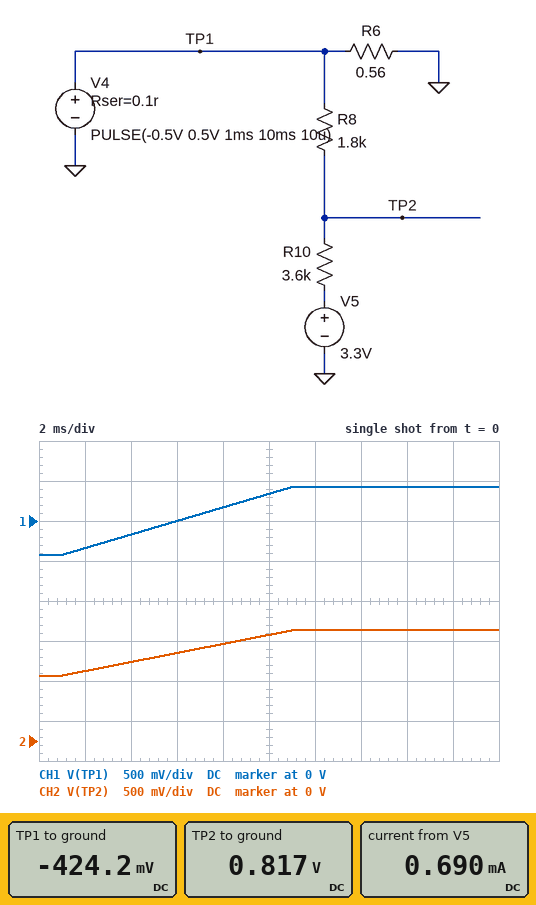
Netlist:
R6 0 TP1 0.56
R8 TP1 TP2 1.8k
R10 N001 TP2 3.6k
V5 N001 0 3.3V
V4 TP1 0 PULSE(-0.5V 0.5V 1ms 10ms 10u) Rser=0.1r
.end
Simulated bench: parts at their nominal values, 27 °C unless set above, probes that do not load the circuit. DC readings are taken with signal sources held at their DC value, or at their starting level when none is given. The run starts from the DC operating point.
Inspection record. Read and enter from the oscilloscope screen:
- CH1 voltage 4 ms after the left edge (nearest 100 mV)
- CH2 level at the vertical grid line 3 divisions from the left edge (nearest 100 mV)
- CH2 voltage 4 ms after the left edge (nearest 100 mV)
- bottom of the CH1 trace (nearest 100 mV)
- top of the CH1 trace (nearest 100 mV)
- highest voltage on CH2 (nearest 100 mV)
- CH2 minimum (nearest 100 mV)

-200 mV
1.1 V
1.0 V
-400 mV
400 mV
1.4 V
800 mV
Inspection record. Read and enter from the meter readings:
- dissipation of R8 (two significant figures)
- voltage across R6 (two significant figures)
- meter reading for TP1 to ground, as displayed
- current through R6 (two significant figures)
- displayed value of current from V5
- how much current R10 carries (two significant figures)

860 µW
420 mV
-424.2 mV
760 mA
0.690 mA
690 µA
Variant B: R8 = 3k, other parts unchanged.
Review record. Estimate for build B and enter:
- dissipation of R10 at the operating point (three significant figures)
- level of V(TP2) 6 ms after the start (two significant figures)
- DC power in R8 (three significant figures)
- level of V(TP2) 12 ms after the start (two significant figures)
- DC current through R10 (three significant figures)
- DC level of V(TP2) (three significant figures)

1.15 mW
1.5 V
955 µW
1.7 V
564 µA
1.27 V
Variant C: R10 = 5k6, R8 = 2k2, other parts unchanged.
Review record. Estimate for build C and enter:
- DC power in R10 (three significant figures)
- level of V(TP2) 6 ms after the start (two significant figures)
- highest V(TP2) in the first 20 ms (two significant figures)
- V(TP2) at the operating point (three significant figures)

1.28 mW
930 mV
1.2 V
626 mV
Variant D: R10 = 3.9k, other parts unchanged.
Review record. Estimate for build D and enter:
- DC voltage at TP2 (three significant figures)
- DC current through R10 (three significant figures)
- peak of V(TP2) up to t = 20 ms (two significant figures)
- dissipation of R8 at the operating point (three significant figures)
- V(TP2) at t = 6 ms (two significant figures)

752 mV
653 µA
1.3 V
768 µW
1.0 V
